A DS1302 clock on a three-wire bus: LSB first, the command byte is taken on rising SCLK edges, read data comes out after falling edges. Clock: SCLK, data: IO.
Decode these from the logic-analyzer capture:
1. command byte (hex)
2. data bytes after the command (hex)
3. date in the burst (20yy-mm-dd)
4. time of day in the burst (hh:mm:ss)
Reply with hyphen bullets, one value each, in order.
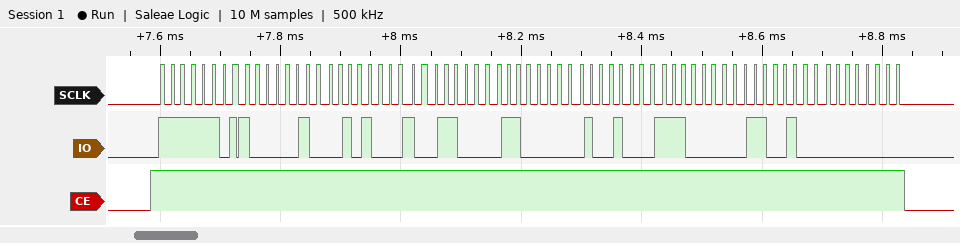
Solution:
- 0xBF
- 41 14 19 06 12 07 26 00
- 2026-12-06
- 19:14:41
